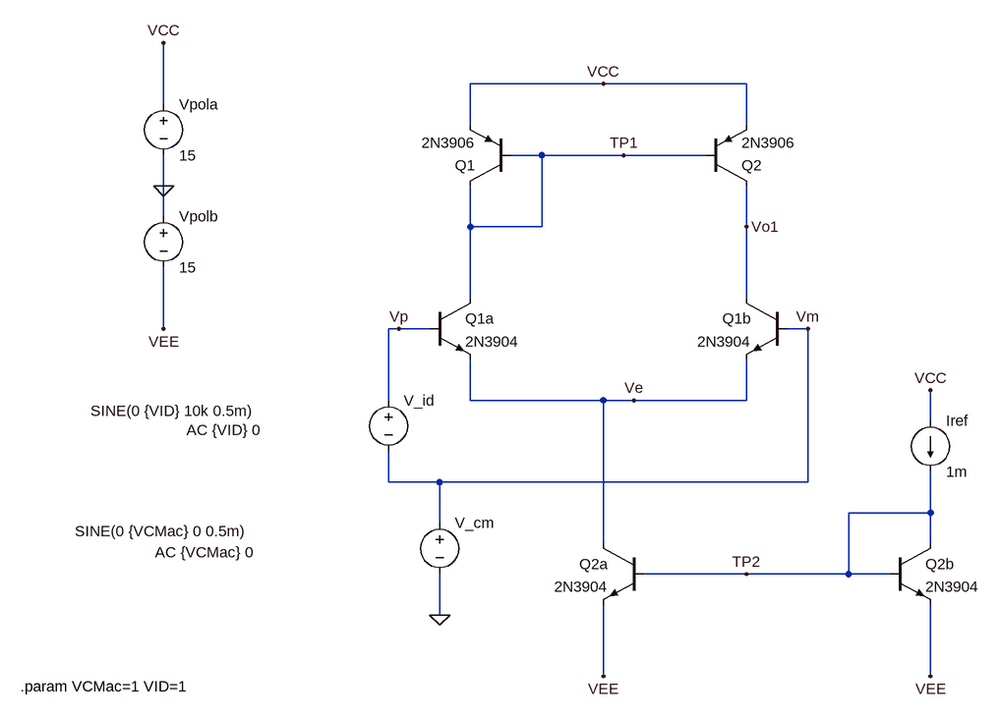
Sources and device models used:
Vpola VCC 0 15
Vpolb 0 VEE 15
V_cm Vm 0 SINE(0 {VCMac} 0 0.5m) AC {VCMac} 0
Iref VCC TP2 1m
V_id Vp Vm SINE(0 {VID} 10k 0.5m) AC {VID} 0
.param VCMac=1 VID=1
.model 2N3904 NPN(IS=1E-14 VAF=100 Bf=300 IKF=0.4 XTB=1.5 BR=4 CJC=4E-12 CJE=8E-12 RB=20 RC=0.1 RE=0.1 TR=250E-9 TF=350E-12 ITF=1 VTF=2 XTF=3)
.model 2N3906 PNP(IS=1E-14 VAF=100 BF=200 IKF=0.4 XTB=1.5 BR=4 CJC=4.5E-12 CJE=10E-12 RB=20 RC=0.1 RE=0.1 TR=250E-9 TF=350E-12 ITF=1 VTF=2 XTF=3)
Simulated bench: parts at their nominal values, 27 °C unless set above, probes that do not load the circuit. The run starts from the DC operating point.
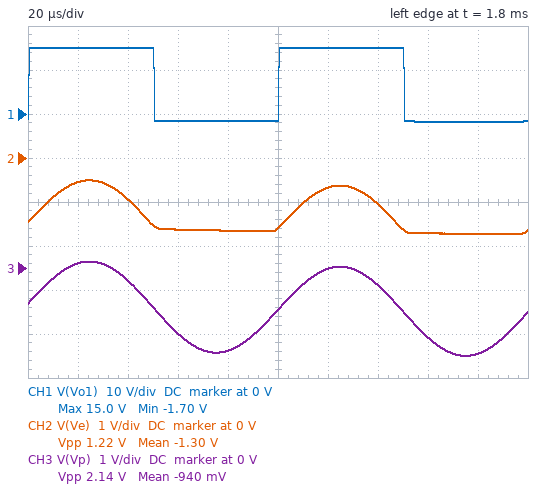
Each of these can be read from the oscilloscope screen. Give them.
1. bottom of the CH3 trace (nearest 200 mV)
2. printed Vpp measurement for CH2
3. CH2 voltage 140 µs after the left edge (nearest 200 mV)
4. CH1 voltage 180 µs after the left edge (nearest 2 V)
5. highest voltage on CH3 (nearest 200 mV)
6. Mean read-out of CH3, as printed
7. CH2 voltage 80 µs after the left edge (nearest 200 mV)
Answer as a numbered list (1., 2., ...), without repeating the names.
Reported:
1. -2.0 V
2. 1.22 V
3. -1.0 V
4. -2 V
5. 200 mV
6. -940 mV
7. -1.6 V
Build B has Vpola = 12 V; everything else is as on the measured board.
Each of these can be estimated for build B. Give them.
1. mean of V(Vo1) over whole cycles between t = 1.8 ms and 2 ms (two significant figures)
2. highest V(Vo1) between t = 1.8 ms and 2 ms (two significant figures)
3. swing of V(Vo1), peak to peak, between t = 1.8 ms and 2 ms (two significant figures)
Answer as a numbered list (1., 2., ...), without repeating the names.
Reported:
1. 5.2 V
2. 12 V
3. 14 V
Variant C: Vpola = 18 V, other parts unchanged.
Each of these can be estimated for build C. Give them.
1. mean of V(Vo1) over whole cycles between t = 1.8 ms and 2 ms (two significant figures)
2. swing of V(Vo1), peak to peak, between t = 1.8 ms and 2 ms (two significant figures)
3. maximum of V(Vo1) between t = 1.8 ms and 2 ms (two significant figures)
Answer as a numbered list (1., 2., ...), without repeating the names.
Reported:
1. 8.2 V
2. 20 V
3. 18 V
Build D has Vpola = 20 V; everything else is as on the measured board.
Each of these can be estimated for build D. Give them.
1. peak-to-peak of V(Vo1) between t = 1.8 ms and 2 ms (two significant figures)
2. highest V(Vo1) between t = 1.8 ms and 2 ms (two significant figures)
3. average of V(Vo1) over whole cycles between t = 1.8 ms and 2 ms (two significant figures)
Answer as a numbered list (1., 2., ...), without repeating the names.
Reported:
1. 22 V
2. 20 V
3. 9.2 V
